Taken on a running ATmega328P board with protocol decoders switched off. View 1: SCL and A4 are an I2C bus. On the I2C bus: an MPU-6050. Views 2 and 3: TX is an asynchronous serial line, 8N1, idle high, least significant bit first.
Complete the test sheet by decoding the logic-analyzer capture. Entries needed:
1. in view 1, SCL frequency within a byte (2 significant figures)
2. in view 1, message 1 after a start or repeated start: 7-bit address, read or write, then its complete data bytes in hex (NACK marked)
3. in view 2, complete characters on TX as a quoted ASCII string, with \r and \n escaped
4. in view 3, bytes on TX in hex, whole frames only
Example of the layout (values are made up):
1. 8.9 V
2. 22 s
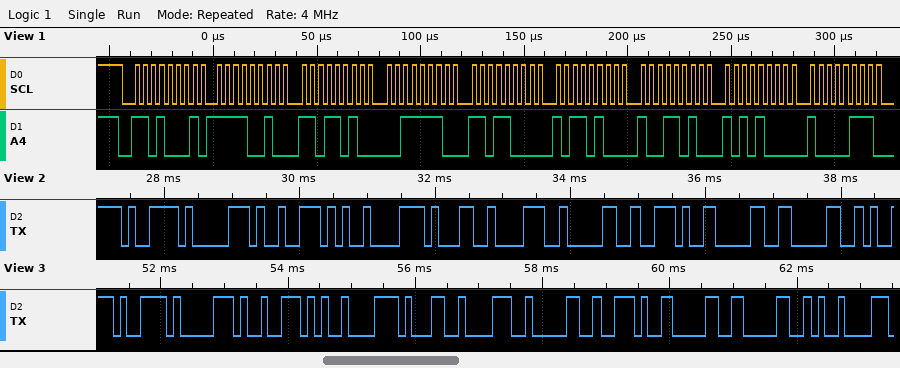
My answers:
1. 250 kHz
2. 0x68 read: F2 DA 3E D8 B4 9A A8 87
3. "ypr\t180.00"
4. 79 70 72 09 31 38 30 2E 30 30 09
